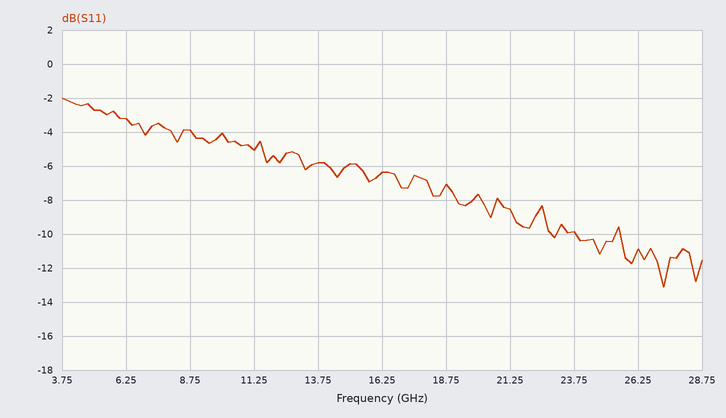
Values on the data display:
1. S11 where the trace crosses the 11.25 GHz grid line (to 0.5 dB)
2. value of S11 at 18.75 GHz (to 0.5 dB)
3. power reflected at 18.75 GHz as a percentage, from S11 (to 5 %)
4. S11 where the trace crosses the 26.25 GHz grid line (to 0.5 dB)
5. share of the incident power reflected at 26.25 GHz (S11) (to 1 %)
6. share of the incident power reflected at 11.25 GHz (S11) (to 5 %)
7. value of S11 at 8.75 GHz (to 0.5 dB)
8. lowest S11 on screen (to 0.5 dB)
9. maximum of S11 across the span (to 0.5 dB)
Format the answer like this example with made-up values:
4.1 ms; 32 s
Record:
-5.0 dB; -7.0 dB; 20 %; -11.0 dB; 8 %; 30 %; -4.0 dB; -13.0 dB; -2.0 dB
